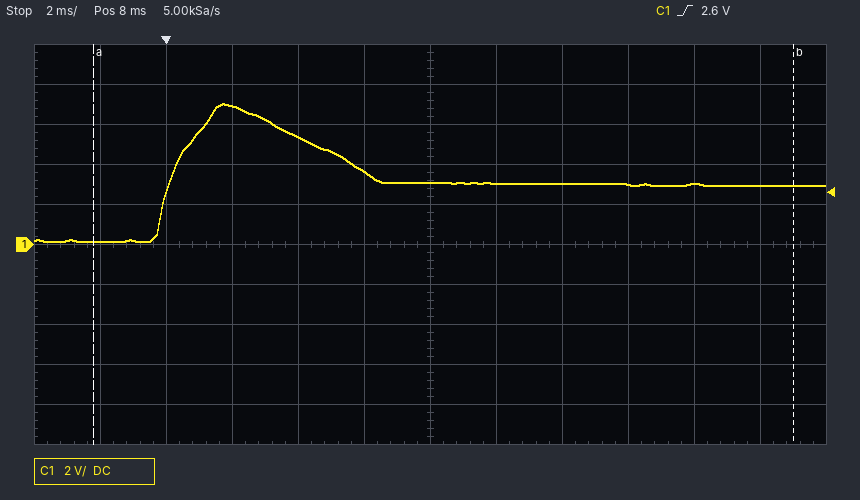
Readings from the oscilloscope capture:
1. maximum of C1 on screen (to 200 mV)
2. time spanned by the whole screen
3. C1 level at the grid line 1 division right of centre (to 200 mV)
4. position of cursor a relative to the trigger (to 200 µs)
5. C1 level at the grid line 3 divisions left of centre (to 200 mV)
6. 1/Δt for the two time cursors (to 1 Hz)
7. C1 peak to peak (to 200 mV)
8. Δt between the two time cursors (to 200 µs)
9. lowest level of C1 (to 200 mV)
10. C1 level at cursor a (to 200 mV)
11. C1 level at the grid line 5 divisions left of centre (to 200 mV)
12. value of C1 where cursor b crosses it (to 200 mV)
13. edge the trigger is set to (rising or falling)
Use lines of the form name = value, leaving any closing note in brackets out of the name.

maximum of C1 on screen = 7.0 V
time spanned by the whole screen = 24 ms
C1 level at the grid line 1 division right of centre = 3.0 V
position of cursor a relative to the trigger = -2.2 ms
C1 level at the grid line 3 divisions left of centre = 7.0 V
1/Δt for the two time cursors = 47 Hz
C1 peak to peak = 6.8 V
Δt between the two time cursors = 21.2 ms
lowest level of C1 = 200 mV
C1 level at cursor a = 200 mV
C1 level at the grid line 5 divisions left of centre = 200 mV
value of C1 where cursor b crosses it = 3.0 V
edge the trigger is set to = rising
